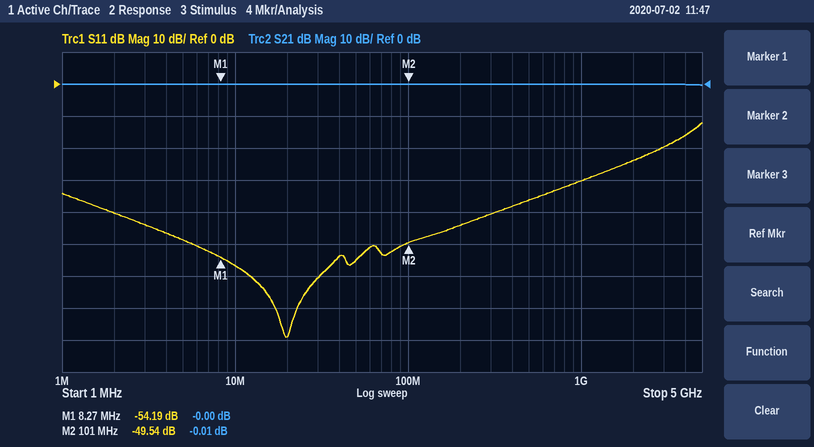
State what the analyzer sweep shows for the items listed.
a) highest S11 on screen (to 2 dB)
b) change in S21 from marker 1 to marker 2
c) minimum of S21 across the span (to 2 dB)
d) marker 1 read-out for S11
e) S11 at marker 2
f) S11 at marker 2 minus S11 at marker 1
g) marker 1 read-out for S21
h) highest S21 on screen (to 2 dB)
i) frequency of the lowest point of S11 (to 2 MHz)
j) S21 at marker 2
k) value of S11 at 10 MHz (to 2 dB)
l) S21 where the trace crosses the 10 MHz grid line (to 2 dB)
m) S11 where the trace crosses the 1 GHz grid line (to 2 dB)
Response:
-12 dB
-0.01 dB
0 dB
-54.19 dB
-49.54 dB
4.65 dB
-0.00 dB
0 dB
20 MHz
-0.01 dB
-56 dB
0 dB
-30 dB
